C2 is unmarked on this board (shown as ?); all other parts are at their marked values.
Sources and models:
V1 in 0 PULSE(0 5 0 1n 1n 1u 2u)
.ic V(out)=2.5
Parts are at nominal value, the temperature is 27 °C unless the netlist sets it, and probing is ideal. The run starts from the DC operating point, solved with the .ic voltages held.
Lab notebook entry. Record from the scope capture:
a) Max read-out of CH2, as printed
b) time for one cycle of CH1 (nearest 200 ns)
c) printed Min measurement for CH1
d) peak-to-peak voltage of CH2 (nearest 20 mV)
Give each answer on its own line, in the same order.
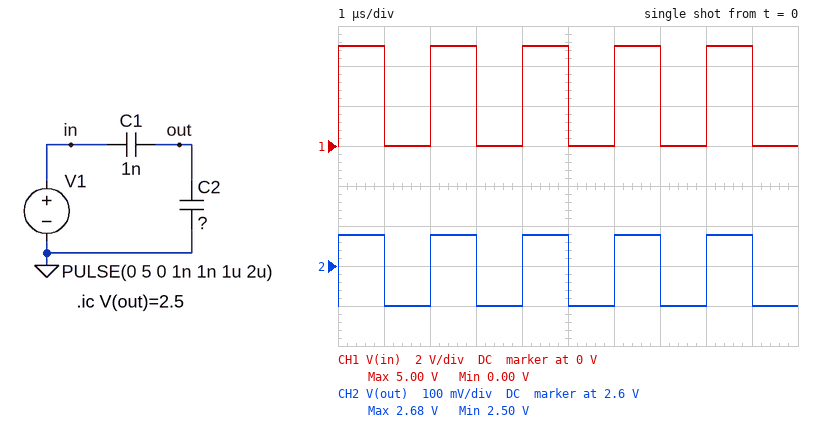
2.68 V
2.0 µs
0.00 V
180 mV
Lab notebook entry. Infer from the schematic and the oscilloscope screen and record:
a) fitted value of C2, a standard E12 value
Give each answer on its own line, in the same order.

27 nF
